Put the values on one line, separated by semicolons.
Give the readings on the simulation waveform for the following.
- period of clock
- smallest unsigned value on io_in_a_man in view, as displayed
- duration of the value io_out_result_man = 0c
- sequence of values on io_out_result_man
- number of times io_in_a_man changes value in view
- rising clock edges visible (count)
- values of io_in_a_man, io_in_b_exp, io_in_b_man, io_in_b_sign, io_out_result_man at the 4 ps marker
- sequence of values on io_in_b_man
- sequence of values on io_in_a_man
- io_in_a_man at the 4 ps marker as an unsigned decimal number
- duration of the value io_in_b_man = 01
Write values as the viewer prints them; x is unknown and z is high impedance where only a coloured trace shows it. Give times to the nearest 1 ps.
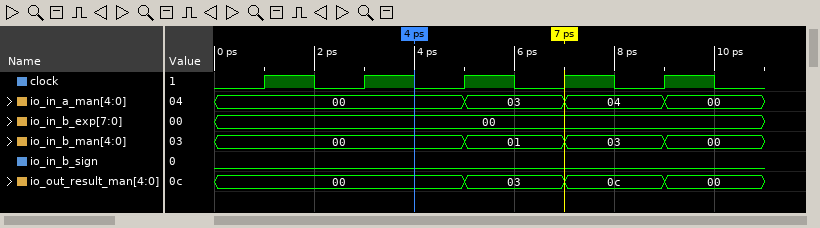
2 ps; 00; 2 ps; 00, 03, 0c, 00; 3; 5; io_in_a_man=00, io_in_b_exp=00, io_in_b_man=00, io_in_b_sign=0, io_out_result_man=00; 00, 01, 03, 00; 00, 03, 04, 00; 0; 2 ps
